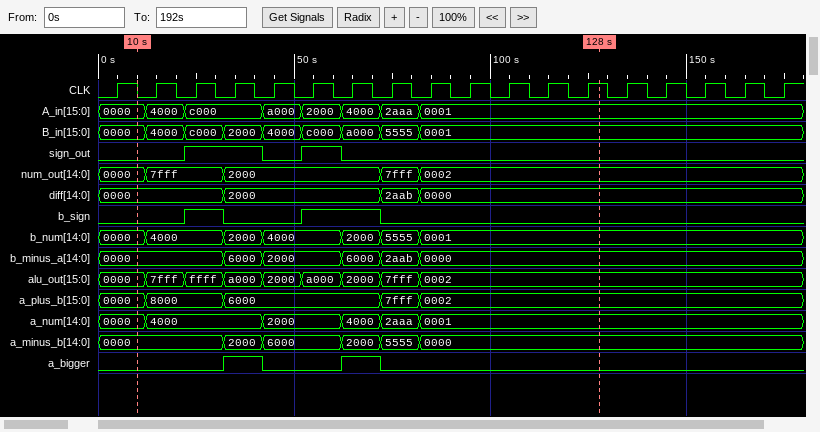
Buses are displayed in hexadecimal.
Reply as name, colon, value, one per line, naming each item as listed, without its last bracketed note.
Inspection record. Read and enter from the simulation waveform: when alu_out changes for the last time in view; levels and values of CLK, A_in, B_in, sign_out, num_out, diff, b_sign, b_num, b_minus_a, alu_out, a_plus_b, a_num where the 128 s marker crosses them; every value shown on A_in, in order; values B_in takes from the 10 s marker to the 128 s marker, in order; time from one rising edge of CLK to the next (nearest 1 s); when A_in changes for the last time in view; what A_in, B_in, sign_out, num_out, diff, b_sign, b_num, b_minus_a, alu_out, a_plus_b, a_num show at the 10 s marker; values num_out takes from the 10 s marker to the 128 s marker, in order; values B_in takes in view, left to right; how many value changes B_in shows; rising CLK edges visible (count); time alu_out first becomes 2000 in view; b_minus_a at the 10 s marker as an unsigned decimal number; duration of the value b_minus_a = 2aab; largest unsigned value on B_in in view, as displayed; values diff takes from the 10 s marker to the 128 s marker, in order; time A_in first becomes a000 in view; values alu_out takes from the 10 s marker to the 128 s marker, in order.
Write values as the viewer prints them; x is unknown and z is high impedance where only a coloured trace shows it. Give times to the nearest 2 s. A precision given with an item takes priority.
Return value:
when alu_out changes for the last time in view: 82 s
levels and values of CLK, A_in, B_in, sign_out, num_out, diff, b_sign, b_num, b_minus_a, alu_out, a_plus_b, a_num where the 128 s marker crosses them: CLK=1, A_in=0001, B_in=0001, sign_out=0, num_out=0002, diff=0000, b_sign=0, b_num=0001, b_minus_a=0000, alu_out=0002, a_plus_b=0002, a_num=0001
every value shown on A_in, in order: 0000, 4000, c000, a000, 2000, 4000, 2aaa, 0001
values B_in takes from the 10 s marker to the 128 s marker, in order: 0000, 4000, c000, 2000, 4000, c000, a000, 5555, 0001
time from one rising edge of CLK to the next: 10 s
when A_in changes for the last time in view: 82 s
what A_in, B_in, sign_out, num_out, diff, b_sign, b_num, b_minus_a, alu_out, a_plus_b, a_num show at the 10 s marker: A_in=0000, B_in=0000, sign_out=0, num_out=0000, diff=0000, b_sign=0, b_num=0000, b_minus_a=0000, alu_out=0000, a_plus_b=0000, a_num=0000
values num_out takes from the 10 s marker to the 128 s marker, in order: 0000, 7fff, 2000, 7fff, 0002
values B_in takes in view, left to right: 0000, 4000, c000, 2000, 4000, c000, a000, 5555, 0001
how many value changes B_in shows: 8
rising CLK edges visible: 18
time alu_out first becomes 2000 in view: 42 s
b_minus_a at the 10 s marker as an unsigned decimal number: 0
duration of the value b_minus_a = 2aab: 10 s
largest unsigned value on B_in in view, as displayed: c000
values diff takes from the 10 s marker to the 128 s marker, in order: 0000, 2000, 2aab, 0000
time A_in first becomes a000 in view: 42 s
values alu_out takes from the 10 s marker to the 128 s marker, in order: 0000, 7fff, ffff, a000, 2000, a000, 2000, 7fff, 0002
